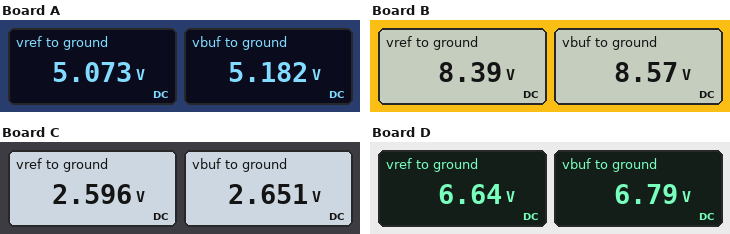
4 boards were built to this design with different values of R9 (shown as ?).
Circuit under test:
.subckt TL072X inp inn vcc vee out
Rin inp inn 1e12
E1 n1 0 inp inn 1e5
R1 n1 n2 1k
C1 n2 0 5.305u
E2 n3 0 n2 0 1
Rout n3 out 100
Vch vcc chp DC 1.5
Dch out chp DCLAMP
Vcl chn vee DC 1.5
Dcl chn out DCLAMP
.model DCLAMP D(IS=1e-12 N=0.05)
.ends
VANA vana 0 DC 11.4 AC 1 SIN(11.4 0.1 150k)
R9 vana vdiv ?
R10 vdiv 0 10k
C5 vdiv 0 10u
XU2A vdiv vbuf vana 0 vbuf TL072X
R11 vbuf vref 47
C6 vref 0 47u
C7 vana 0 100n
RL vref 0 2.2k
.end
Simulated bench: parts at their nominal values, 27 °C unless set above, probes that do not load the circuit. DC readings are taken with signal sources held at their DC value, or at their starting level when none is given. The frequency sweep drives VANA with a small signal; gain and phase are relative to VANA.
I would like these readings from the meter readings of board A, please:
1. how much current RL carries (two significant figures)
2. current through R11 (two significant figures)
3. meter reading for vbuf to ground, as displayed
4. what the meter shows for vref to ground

2.3 mA
2.3 mA
5.182 V
5.073 V
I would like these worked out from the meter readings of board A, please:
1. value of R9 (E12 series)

12 kΩ
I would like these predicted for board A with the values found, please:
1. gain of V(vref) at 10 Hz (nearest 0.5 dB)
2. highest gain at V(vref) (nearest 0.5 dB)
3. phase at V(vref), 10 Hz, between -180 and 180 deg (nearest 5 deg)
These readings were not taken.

-18.0 dB
-7.0 dB
-80 deg
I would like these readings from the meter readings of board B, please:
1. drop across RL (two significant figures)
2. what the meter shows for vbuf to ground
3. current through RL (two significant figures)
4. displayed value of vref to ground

8.4 V
8.57 V
3.8 mA
8.39 V
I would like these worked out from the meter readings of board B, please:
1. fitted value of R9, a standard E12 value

3.3 kΩ
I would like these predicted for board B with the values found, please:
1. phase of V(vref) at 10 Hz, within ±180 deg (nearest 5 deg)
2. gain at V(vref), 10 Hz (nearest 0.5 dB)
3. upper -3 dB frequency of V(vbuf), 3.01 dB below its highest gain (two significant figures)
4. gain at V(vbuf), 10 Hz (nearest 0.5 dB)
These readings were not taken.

-65 deg
-8.0 dB
6.4 Hz
-8.0 dB
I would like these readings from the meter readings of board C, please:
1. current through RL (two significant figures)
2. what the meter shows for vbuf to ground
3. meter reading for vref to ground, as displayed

1.2 mA
2.651 V
2.596 V
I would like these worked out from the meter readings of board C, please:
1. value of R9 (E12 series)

33 kΩ
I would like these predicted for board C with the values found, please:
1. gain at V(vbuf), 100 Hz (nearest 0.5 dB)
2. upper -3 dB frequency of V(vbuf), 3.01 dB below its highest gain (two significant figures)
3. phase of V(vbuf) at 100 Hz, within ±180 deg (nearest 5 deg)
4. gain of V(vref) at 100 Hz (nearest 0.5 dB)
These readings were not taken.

-46.5 dB
2.1 Hz
-90 deg
-51.0 dB
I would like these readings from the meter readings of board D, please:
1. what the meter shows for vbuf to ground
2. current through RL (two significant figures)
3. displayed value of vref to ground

6.79 V
3.0 mA
6.64 V
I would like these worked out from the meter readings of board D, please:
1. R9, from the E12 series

6.8 kΩ
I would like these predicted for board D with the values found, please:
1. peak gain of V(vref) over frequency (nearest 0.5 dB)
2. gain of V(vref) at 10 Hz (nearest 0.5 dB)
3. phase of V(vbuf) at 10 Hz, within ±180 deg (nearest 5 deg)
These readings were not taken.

-4.5 dB
-13.5 dB
-70 deg
